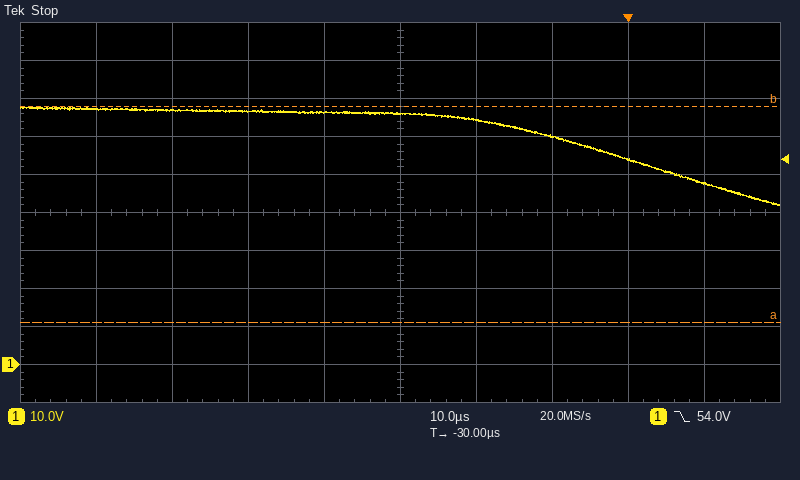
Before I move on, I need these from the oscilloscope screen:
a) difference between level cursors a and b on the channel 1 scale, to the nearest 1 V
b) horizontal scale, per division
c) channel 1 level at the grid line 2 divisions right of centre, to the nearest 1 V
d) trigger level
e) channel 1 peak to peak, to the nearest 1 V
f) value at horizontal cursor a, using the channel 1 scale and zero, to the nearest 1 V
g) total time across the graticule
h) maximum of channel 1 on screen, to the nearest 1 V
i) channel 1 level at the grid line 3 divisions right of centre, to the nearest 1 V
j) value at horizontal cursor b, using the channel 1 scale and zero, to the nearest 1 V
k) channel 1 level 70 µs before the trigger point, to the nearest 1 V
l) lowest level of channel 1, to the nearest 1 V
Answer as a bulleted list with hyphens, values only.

- 57 V
- 10 µs
- 60 V
- 54.0 V
- 26 V
- 11 V
- 100 µs
- 68 V
- 54 V
- 68 V
- 67 V
- 42 V
